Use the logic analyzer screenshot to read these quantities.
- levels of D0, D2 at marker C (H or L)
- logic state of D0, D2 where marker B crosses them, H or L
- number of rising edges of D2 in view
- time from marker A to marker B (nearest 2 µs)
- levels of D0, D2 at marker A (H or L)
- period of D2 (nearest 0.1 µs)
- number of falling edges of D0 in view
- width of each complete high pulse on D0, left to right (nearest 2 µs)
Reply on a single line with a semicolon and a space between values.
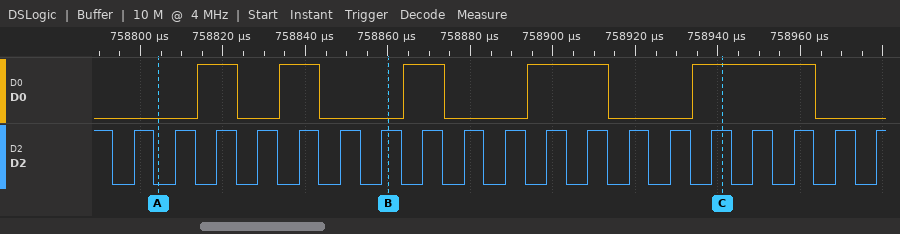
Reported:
D0=H, D2=H; D0=L, D2=H; 19; 56 µs; D0=L, D2=L; 10 µs; 5; 10 µs, 10 µs, 10 µs, 20 µs, 30 µs
